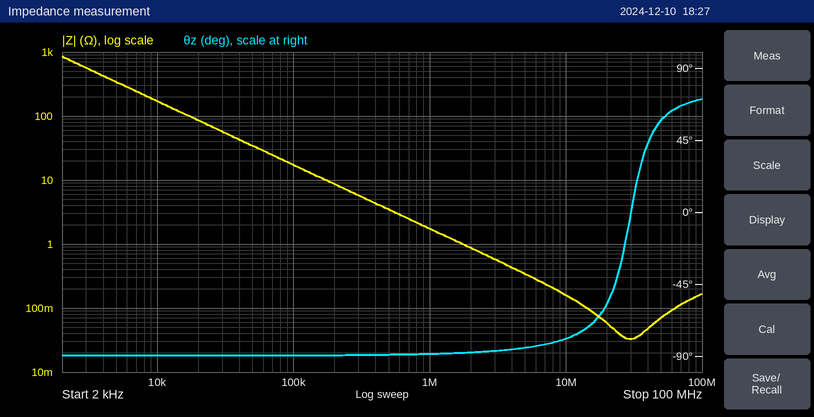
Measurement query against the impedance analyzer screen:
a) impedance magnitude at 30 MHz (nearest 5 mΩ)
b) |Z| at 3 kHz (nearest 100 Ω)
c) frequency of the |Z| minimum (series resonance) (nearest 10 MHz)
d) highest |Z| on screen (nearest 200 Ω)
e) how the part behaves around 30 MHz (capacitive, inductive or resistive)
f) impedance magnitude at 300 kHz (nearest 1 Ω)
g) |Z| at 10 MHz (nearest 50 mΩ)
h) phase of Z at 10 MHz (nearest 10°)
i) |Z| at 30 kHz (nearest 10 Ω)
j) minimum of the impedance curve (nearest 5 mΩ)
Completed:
35 mΩ
600 Ω
30 MHz
800 Ω
resistive
6 Ω
150 mΩ
-80°
60 Ω
35 mΩ
